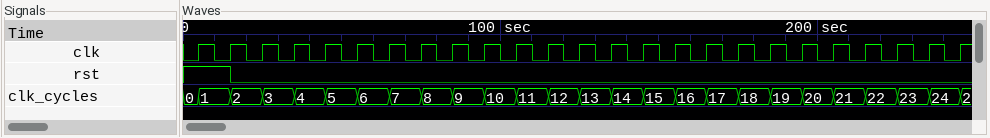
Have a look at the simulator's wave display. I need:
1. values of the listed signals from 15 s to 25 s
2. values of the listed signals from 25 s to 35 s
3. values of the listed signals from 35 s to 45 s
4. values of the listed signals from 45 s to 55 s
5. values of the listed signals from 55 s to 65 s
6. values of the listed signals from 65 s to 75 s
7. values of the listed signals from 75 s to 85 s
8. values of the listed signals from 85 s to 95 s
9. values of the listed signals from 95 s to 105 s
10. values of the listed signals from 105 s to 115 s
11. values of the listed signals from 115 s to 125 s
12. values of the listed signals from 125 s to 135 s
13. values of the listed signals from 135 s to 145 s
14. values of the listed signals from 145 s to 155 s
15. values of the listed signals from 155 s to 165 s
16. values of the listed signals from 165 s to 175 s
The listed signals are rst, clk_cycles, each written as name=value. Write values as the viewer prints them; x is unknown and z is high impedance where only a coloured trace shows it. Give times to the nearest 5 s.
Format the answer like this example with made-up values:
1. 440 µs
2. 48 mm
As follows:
1. rst=0, clk_cycles=2
2. rst=0, clk_cycles=3
3. rst=0, clk_cycles=4
4. rst=0, clk_cycles=5
5. rst=0, clk_cycles=6
6. rst=0, clk_cycles=7
7. rst=0, clk_cycles=8
8. rst=0, clk_cycles=9
9. rst=0, clk_cycles=10
10. rst=0, clk_cycles=11
11. rst=0, clk_cycles=12
12. rst=0, clk_cycles=13
13. rst=0, clk_cycles=14
14. rst=0, clk_cycles=15
15. rst=0, clk_cycles=16
16. rst=0, clk_cycles=17
